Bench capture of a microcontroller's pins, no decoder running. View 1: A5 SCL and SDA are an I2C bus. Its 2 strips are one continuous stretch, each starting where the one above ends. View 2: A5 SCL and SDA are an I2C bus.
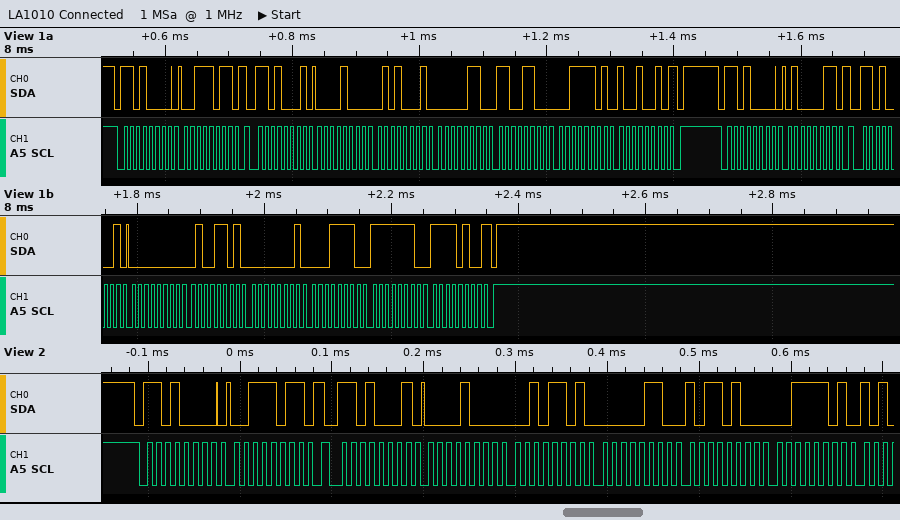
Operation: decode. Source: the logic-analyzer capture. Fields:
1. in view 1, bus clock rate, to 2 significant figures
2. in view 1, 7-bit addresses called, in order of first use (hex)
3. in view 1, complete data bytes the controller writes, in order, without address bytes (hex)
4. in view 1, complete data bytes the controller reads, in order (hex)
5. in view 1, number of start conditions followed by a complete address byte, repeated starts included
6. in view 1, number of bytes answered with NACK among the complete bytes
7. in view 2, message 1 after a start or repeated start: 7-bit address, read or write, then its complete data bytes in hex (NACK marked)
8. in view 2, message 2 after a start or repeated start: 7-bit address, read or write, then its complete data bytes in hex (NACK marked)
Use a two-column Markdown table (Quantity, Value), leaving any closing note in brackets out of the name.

| Quantity | Value |
|---|---|
| in view 1, bus clock rate, to 2 significant figures | 100 kHz |
| in view 1, 7-bit addresses called, in order of first use | 0x68 |
| in view 1, complete data bytes the controller writes, in order, without address bytes | 3B 43 |
| in view 1, complete data bytes the controller reads, in order | 08 51 06 CC 3D 92 00 4D 01 1E FE F4 |
| in view 1, number of start conditions followed by a complete address byte, repeated starts included | 4 |
| in view 1, number of bytes answered with NACK among the complete bytes | 2 |
| in view 2, message 1 after a start or repeated start: 7-bit address, read or write, then its complete data bytes in hex | 0x68 write: 3B |
| in view 2, message 2 after a start or repeated start: 7-bit address, read or write, then its complete data bytes in hex | 0x68 read: 08 2D 06 B4 3D |
